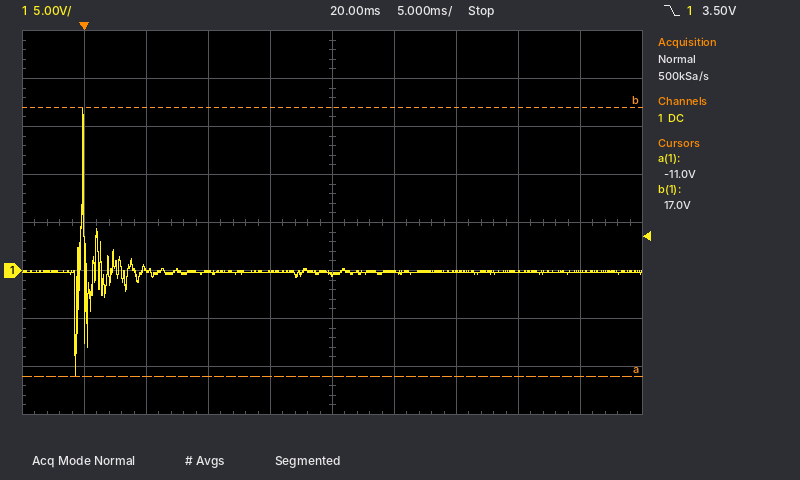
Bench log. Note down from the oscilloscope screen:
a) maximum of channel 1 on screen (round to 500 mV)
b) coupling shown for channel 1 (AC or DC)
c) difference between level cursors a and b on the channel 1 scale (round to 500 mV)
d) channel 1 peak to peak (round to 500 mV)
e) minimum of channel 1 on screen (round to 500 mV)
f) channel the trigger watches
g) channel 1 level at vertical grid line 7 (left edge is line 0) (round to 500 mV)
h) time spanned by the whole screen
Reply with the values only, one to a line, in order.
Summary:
17.0 V
DC
28.0 V
28.0 V
-11.0 V
channel 1
0.0 V
50 ms
